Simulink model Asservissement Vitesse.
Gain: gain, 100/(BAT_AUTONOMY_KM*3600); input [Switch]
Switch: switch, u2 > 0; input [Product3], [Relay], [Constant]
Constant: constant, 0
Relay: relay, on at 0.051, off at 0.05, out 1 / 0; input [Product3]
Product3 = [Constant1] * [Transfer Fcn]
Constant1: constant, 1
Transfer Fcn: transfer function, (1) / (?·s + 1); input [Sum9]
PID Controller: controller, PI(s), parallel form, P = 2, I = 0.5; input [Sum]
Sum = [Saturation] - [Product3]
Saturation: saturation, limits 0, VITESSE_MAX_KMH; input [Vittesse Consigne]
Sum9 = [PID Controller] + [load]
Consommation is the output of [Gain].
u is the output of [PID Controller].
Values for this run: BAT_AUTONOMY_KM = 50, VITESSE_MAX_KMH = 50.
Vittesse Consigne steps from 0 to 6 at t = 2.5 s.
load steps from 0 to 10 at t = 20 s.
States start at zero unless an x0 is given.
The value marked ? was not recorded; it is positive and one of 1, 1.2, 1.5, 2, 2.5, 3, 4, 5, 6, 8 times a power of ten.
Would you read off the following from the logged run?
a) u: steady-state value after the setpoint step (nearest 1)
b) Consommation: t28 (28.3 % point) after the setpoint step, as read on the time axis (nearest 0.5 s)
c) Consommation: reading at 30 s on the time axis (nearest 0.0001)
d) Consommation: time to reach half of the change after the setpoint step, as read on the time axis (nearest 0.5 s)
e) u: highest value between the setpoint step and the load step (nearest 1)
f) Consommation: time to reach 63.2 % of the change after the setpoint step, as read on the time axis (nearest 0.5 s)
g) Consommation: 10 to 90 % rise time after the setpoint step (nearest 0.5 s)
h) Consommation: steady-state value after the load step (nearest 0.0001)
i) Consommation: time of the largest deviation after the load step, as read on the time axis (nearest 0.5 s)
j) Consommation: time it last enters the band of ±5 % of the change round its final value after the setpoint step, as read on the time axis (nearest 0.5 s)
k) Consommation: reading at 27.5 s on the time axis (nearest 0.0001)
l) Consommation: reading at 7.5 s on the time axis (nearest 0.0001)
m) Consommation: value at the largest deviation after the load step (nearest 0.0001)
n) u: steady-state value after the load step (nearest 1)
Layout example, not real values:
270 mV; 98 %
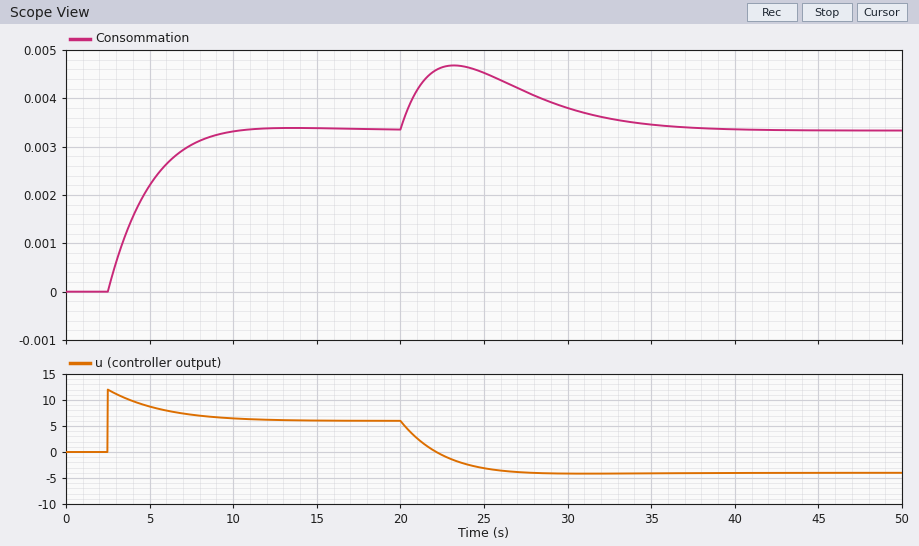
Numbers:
6; 3.5 s; 0.0038; 4.0 s; 12; 5.0 s; 4.5 s; 0.0033; 23.0 s; 8.5 s; 0.0041; 0.0030; 0.0047; -4
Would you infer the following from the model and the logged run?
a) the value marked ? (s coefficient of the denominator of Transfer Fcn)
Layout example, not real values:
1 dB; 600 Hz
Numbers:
5
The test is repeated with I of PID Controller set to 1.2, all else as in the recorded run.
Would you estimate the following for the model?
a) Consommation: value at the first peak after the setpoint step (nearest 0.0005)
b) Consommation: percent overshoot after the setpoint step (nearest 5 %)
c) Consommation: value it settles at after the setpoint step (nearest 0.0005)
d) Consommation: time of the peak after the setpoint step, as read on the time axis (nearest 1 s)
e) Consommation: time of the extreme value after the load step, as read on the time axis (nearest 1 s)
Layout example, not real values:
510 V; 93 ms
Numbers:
0.0040; 15 %; 0.0035; 8 s; 22 s
